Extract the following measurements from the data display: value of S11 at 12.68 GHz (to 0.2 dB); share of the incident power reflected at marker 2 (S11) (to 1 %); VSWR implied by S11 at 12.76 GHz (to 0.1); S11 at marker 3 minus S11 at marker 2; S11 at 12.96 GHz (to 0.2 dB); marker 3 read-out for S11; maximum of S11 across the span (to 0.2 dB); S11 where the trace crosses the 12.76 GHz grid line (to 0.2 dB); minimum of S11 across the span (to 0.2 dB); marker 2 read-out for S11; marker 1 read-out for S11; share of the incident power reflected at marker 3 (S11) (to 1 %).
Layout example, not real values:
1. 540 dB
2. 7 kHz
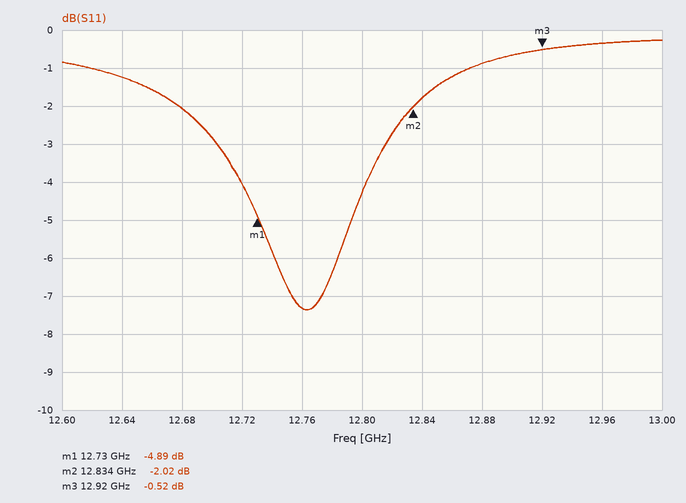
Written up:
1. -2.0 dB
2. 63 %
3. 2.5
4. 1.50 dB
5. -0.4 dB
6. -0.52 dB
7. -0.2 dB
8. -7.4 dB
9. -7.4 dB
10. -2.02 dB
11. -4.89 dB
12. 89 %
